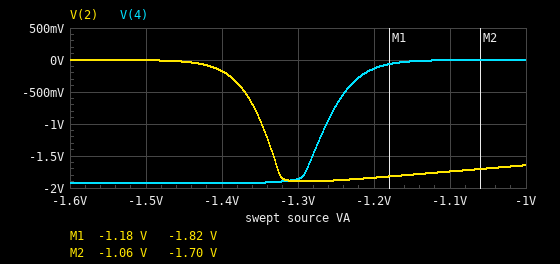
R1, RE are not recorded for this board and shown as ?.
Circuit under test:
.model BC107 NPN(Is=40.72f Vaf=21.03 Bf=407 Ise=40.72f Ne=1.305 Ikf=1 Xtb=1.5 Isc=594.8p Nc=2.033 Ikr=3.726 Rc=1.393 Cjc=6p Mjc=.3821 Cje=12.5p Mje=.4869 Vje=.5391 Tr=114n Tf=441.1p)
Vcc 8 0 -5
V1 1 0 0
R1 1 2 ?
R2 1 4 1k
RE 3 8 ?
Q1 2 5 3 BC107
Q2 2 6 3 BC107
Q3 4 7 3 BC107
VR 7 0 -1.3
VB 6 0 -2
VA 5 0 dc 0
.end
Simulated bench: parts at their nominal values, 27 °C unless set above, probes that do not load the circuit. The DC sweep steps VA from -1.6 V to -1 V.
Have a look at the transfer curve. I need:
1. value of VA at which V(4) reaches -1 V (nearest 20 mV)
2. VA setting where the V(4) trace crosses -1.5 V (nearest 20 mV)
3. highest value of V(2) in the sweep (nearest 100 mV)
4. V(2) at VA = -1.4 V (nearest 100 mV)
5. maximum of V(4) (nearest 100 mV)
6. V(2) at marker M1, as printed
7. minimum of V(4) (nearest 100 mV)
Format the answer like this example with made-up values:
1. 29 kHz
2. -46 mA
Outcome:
1. -1.26 V
2. -1.28 V
3. 0 V
4. -200 mV
5. 0 V
6. -1.82 V
7. -1.9 V
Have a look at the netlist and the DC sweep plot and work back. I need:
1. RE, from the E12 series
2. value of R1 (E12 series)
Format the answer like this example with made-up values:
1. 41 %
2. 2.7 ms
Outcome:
1. 820 Ω
2. 1.5 kΩ
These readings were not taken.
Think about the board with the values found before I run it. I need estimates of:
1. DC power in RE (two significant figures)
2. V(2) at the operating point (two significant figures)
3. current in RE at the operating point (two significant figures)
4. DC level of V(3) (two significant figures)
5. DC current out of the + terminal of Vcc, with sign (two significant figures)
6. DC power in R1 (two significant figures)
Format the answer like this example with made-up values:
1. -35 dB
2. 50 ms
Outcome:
1. 23 mW
2. -660 mV
3. 5.3 mA
4. -680 mV
5. -5.3 mA
6. 290 µW
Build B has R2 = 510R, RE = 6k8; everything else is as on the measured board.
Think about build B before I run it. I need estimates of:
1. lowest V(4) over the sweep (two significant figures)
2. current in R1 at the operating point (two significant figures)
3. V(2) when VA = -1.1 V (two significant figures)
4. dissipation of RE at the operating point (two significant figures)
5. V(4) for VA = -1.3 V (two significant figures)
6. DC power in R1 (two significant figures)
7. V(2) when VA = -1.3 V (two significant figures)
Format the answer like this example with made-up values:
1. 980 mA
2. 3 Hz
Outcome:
1. -230 mV
2. 390 µA
3. -720 mV
4. 2.8 mW
5. -120 mV
6. 220 µW
7. -340 mV
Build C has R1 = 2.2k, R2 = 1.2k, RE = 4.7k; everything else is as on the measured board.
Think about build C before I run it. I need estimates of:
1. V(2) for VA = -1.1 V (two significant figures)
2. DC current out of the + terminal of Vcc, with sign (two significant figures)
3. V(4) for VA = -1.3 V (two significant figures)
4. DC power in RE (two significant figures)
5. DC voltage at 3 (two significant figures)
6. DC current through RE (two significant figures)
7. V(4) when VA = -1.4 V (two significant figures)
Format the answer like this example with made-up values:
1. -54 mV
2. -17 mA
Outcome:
1. -1.5 V
2. -930 µA
3. -400 mV
4. 4.1 mW
5. -630 mV
6. 930 µA
7. -770 mV
